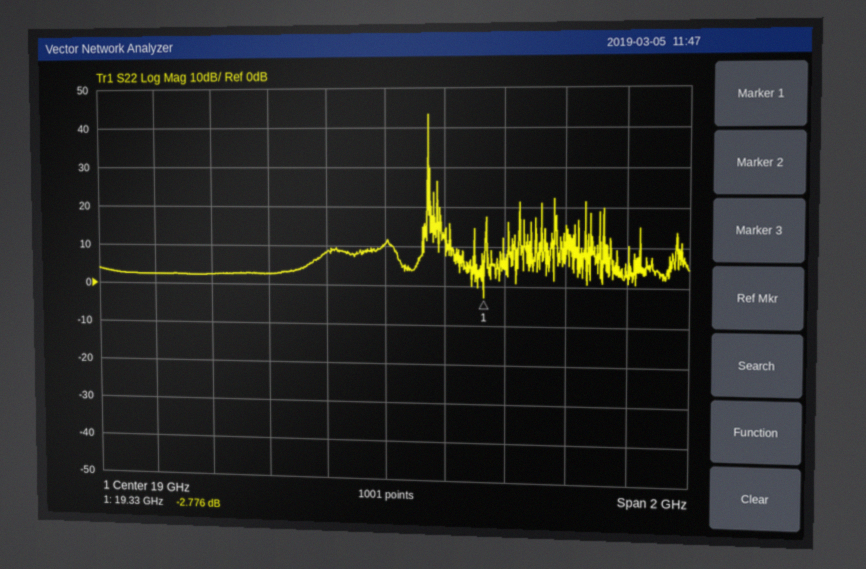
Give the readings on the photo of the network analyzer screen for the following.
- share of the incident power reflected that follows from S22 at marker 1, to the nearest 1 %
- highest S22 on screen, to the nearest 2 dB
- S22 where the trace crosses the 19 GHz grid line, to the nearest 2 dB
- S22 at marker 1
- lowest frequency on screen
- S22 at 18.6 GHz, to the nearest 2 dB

53 %
44 dB
10 dB
-2.776 dB
18 GHz
2 dB
